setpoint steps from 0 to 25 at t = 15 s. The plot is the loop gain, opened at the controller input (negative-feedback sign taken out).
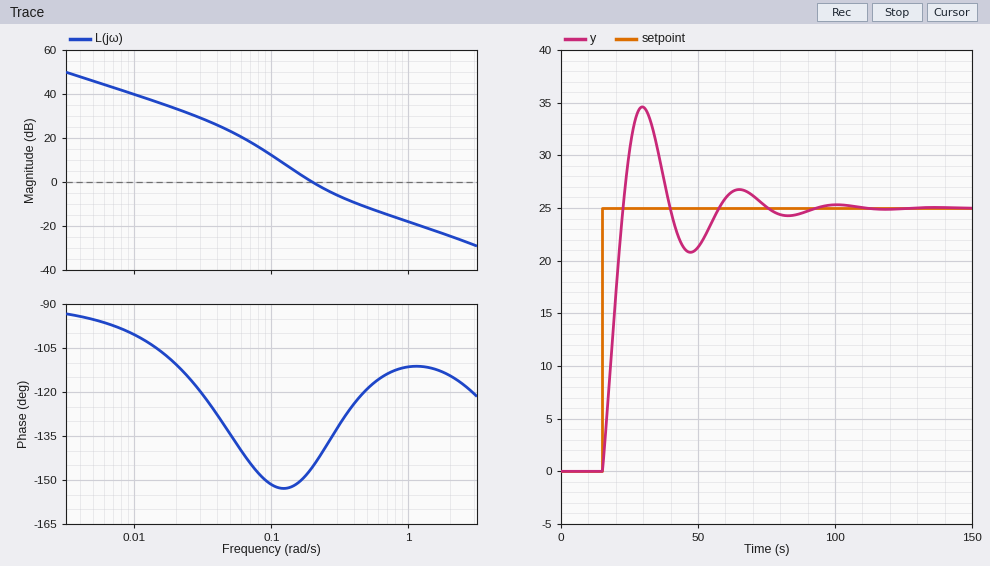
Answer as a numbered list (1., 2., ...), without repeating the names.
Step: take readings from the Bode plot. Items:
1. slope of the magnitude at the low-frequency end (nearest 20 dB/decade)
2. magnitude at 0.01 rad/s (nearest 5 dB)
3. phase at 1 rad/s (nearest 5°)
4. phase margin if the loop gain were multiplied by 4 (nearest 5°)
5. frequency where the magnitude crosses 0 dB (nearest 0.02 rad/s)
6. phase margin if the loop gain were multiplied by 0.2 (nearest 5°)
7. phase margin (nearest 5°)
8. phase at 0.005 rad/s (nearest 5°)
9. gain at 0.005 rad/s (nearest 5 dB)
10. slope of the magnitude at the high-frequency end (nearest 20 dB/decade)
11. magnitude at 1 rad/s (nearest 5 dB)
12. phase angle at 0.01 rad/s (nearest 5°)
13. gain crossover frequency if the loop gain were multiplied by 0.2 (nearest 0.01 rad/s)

1. -20 dB/decade
2. 40 dB
3. -110°
4. 60°
5. 0.20 rad/s
6. 30°
7. 35°
8. -95°
9. 45 dB
10. -20 dB/decade
11. -20 dB
12. -100°
13. 0.09 rad/s
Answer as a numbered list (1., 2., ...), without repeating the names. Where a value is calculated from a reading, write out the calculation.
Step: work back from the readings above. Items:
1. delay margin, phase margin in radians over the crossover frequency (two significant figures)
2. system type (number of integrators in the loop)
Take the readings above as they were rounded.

1. 35 × π / 180 / 0.2 = 3.1 s
2. 1
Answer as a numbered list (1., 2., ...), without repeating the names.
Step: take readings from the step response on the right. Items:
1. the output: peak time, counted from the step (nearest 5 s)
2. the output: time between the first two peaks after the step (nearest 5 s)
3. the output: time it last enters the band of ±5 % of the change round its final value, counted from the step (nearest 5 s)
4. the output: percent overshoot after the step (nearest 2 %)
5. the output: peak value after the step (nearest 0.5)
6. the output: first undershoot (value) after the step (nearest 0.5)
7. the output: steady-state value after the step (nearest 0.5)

1. 15 s
2. 35 s
3. 55 s
4. 38 %
5. 34.5
6. 21.0
7. 25.0
